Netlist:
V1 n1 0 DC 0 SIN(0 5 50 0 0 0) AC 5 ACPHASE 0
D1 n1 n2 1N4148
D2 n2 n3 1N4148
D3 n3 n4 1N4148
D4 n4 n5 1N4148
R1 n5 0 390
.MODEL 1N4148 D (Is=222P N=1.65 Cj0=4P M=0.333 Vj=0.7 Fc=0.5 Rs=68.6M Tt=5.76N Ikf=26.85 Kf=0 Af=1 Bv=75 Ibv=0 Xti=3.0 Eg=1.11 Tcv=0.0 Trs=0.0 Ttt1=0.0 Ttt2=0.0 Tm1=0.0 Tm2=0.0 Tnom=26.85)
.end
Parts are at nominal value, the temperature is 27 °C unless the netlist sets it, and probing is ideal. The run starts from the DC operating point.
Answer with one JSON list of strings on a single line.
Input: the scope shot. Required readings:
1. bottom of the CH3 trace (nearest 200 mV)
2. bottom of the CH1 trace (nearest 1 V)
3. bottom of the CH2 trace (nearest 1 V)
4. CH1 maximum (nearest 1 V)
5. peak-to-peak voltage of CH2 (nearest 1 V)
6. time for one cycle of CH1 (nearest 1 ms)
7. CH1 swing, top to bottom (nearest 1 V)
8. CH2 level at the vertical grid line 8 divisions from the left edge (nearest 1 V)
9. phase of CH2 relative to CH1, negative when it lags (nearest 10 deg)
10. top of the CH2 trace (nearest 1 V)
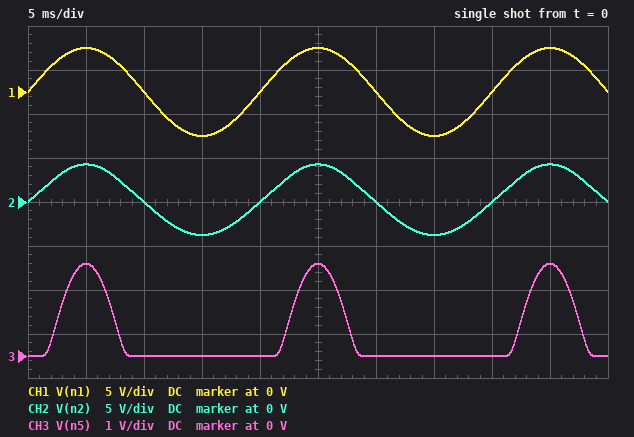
["0 V", "-5 V", "-4 V", "5 V", "8 V", "20 ms", "10 V", "0 V", "0 deg", "4 V"]
